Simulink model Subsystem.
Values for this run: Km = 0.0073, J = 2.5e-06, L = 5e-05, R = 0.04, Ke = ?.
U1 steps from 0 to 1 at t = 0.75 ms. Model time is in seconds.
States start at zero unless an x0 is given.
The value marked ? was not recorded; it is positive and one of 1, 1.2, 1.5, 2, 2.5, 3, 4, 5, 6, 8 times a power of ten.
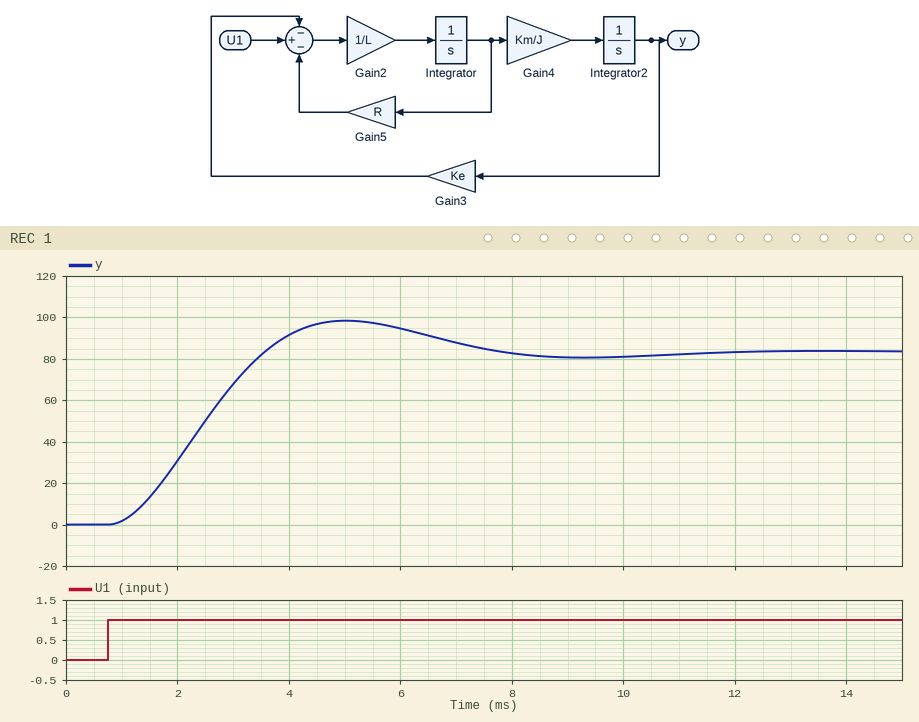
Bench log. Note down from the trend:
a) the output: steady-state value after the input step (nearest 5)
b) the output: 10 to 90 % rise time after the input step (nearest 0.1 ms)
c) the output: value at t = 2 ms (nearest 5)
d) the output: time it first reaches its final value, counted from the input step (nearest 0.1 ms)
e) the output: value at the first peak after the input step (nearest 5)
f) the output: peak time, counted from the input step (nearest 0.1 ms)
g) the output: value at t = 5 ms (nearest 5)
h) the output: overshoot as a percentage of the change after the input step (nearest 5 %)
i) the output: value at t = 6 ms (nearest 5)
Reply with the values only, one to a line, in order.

85
1.9 ms
30
2.8 ms
100
4.3 ms
100
20 %
95
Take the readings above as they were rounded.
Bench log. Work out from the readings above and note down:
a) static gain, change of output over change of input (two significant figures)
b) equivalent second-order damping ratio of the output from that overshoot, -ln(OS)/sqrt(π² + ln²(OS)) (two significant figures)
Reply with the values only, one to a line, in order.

85
0.46
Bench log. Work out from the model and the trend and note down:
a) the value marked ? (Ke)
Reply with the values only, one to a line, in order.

0.012
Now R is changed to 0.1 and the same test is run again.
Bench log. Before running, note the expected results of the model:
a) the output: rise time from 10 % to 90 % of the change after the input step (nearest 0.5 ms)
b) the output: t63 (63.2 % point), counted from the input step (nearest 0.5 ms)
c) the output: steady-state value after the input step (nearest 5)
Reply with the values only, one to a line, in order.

5.0 ms
3.0 ms
85
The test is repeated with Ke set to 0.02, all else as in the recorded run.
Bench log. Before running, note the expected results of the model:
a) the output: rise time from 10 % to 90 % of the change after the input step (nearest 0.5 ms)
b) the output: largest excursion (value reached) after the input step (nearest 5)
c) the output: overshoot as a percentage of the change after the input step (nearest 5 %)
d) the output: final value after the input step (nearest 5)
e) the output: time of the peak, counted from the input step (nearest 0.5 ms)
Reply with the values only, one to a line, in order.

1.5 ms
65
30 %
50
3.0 ms
